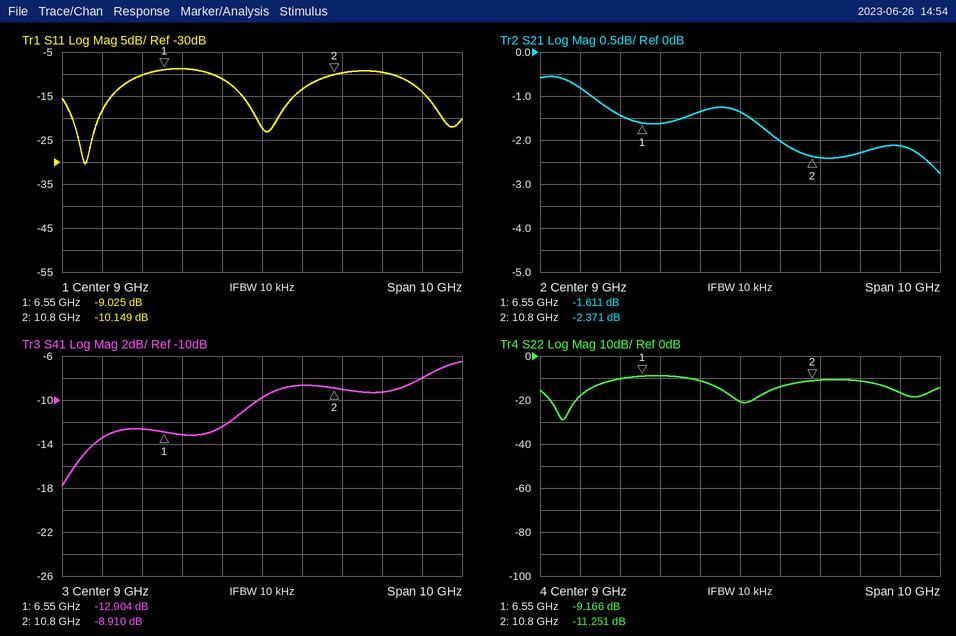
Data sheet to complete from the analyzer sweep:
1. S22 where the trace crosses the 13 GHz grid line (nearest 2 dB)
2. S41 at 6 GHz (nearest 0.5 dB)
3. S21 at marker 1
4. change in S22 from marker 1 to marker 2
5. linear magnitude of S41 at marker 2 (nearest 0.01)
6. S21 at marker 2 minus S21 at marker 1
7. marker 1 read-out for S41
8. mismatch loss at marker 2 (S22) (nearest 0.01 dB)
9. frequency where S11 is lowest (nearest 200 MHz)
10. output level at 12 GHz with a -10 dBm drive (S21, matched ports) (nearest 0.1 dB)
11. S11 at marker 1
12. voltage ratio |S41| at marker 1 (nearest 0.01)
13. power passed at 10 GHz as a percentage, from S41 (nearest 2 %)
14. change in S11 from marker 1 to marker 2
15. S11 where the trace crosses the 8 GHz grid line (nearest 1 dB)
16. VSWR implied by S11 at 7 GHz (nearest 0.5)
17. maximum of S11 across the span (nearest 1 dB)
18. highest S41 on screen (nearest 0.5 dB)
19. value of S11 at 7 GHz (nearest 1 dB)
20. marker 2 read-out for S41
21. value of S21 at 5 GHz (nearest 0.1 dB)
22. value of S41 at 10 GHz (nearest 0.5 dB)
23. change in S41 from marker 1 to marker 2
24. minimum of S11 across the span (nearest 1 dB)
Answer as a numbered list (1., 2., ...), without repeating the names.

1. -16 dB
2. -12.5 dB
3. -1.611 dB
4. -2.085 dB
5. 0.36
6. -0.760 dB
7. -12.904 dB
8. 0.34 dB
9. 4.6 GHz
10. -12.3 dBm
11. -9.025 dB
12. 0.23
13. 14 %
14. -1.124 dB
15. -11 dB
16. 2.0
17. -9 dB
18. -6.5 dB
19. -9 dB
20. -8.910 dB
21. -0.8 dB
22. -8.5 dB
23. 3.994 dB
24. -30 dB
